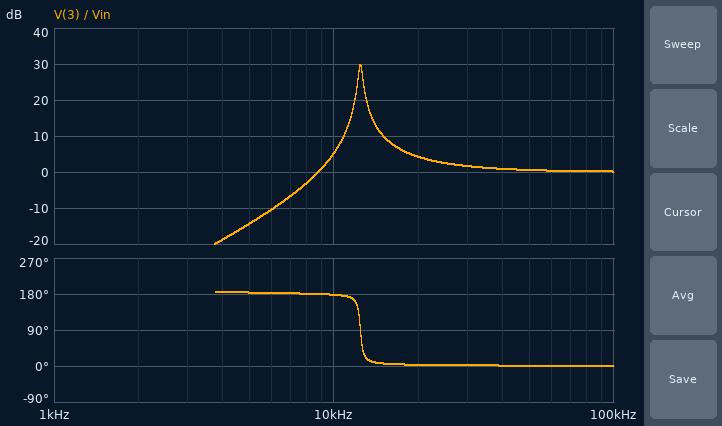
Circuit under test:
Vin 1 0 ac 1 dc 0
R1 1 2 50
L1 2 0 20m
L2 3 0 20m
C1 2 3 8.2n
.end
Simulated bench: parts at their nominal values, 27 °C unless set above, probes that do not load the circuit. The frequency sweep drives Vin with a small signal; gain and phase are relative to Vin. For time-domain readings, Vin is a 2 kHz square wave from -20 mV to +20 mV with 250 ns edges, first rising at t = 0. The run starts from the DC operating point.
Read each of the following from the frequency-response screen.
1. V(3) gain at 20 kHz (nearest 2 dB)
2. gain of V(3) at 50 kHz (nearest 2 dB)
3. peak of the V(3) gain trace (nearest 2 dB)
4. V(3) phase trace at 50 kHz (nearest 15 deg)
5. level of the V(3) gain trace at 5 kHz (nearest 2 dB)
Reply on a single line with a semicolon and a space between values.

4 dB; 0 dB; 30 dB; 0 deg; -14 dB
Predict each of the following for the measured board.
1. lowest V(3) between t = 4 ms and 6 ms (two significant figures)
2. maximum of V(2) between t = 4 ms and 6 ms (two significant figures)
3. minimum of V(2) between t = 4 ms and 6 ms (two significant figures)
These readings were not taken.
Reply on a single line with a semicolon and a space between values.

-24 mV; 26 mV; -26 mV
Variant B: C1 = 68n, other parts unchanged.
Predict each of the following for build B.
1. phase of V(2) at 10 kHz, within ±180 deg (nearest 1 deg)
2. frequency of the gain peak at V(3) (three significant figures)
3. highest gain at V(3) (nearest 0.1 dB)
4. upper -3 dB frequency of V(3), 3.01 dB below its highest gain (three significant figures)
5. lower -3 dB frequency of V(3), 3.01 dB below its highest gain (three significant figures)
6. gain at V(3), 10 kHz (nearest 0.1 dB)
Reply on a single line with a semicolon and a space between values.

5 deg; 4.31 kHz; 20.7 dB; 4.52 kHz; 4.12 kHz; 1.8 dB
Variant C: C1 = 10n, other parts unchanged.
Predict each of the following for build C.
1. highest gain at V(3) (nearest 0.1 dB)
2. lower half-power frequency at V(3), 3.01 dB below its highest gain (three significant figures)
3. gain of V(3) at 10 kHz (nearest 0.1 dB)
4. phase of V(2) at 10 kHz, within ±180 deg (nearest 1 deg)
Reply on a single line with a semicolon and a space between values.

29.0 dB; 11.1 kHz; 11.4 dB; -6 deg
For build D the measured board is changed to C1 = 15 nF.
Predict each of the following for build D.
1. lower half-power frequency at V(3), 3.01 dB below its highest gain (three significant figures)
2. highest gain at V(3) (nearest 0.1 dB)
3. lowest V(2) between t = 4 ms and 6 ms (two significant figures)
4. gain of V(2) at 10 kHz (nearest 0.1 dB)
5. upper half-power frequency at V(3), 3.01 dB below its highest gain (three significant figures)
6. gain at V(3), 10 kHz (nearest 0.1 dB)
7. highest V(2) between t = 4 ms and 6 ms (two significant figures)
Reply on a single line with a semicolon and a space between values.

8.99 kHz; 27.3 dB; -27 mV; -0.4 dB; 9.39 kHz; 15.8 dB; 27 mV
